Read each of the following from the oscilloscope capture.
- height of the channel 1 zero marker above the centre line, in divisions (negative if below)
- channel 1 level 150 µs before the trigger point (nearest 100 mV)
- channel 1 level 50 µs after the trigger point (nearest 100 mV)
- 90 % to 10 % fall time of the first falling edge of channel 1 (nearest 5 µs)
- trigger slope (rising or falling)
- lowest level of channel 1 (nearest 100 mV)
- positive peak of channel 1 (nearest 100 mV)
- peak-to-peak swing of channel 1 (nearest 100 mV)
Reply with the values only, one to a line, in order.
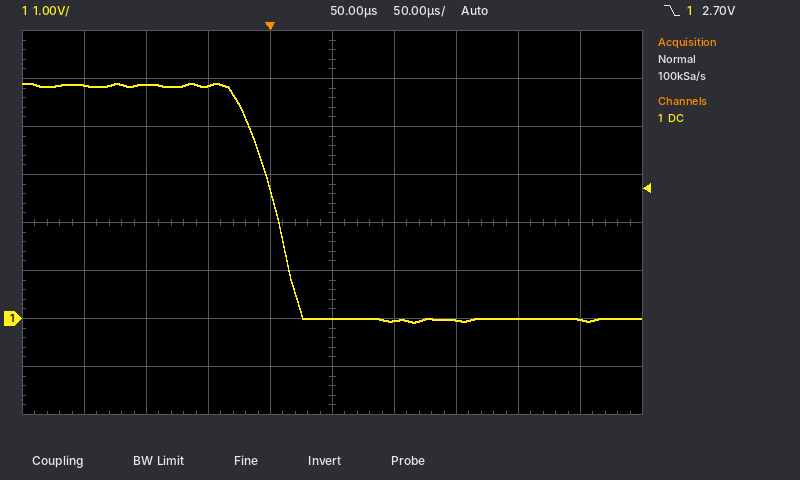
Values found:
-2.0 div
4.9 V
0.0 V
45 µs
falling
-100 mV
4.9 V
5.0 V
